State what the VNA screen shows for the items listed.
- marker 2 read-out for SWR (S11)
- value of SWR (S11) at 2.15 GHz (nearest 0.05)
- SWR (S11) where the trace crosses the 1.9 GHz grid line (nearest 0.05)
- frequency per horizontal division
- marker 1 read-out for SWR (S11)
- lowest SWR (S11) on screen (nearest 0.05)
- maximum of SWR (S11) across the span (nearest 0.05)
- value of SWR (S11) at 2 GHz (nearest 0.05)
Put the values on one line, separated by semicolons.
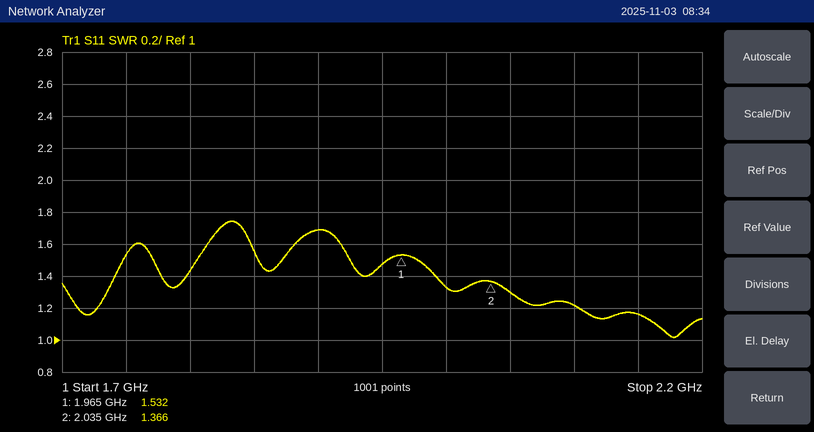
1.366; 1.15; 1.70; 50 MHz; 1.532; 1.00; 1.75; 1.35
